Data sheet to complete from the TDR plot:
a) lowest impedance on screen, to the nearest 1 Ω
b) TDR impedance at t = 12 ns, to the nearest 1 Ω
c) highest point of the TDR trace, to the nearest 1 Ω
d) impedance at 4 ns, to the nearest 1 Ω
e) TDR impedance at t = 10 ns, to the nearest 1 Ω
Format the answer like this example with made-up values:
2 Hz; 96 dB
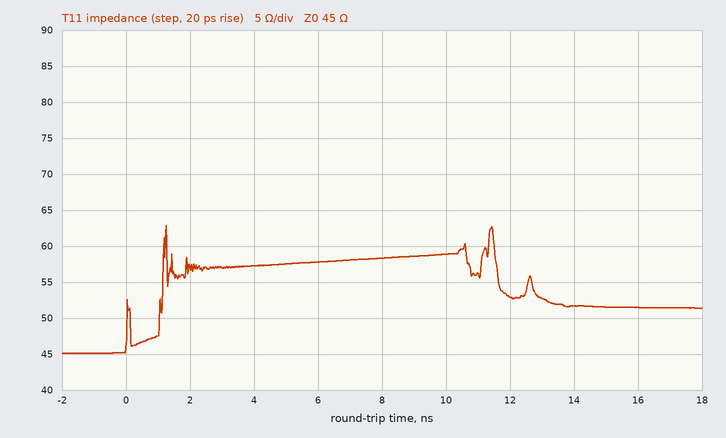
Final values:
45 Ω; 53 Ω; 63 Ω; 57 Ω; 59 Ω
